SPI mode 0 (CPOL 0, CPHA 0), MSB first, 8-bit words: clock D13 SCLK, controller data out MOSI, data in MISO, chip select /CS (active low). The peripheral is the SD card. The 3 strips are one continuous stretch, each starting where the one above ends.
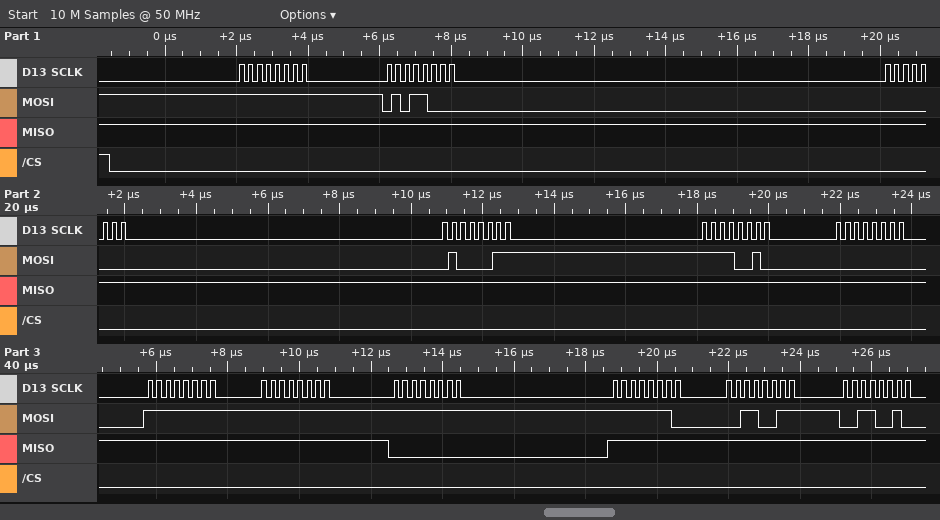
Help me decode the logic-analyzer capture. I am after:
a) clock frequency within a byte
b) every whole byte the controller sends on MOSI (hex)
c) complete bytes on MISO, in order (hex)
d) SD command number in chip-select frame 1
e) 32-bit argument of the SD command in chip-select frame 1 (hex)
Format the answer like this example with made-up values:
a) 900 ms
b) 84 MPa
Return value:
a) 4 MHz
b) FF 58 00 43 F2 00 FF FF FF FE 33 32
c) FF FF FF FF FF FF FF FF 00 FF FF FF
d) CMD24
e) 0x0043F200
